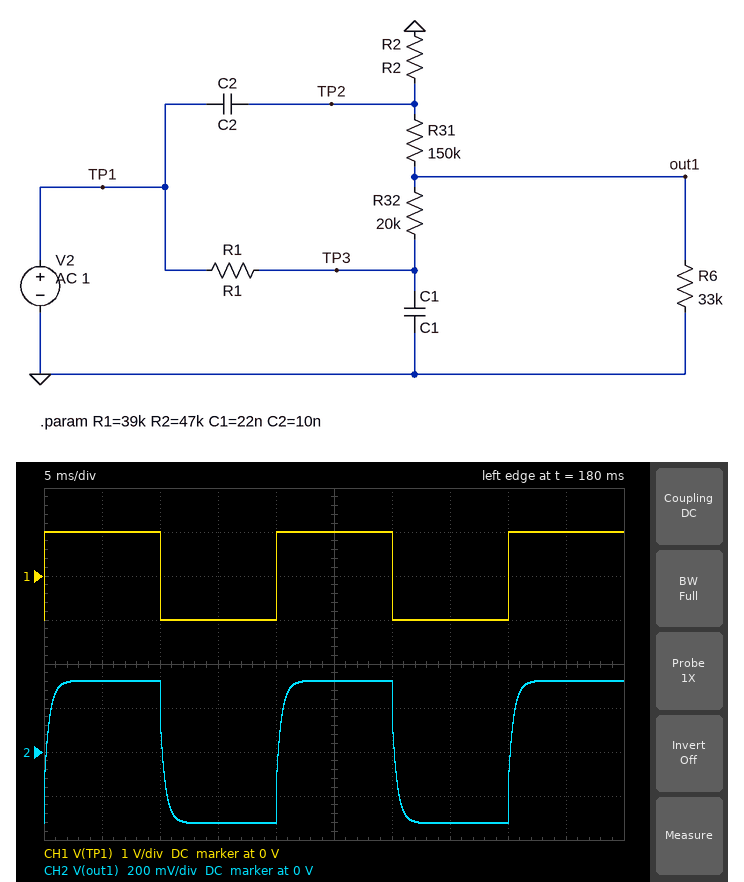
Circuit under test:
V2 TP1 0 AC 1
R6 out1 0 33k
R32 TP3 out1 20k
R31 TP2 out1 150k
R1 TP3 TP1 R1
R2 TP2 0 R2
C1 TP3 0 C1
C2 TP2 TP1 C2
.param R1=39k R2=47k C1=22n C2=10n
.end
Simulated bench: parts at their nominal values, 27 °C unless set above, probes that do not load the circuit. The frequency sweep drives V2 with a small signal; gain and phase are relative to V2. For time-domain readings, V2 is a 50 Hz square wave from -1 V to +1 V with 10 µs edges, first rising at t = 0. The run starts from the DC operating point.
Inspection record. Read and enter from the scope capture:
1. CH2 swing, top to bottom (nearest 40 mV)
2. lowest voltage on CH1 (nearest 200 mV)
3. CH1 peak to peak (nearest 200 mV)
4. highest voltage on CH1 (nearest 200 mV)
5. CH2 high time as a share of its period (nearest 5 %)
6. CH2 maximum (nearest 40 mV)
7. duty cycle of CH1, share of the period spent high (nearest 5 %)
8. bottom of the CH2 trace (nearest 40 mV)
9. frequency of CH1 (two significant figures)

640 mV
-1.0 V
2.0 V
1.0 V
50 %
320 mV
50 %
-320 mV
50 Hz
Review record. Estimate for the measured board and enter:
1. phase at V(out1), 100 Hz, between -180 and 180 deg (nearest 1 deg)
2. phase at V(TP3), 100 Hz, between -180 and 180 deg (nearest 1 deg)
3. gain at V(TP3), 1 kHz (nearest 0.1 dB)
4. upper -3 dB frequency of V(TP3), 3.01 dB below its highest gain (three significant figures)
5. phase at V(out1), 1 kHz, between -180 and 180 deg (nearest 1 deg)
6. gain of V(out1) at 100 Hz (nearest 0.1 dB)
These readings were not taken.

-12 deg
-15 deg
-14.1 dB
375 Hz
-37 deg
-10.1 dB
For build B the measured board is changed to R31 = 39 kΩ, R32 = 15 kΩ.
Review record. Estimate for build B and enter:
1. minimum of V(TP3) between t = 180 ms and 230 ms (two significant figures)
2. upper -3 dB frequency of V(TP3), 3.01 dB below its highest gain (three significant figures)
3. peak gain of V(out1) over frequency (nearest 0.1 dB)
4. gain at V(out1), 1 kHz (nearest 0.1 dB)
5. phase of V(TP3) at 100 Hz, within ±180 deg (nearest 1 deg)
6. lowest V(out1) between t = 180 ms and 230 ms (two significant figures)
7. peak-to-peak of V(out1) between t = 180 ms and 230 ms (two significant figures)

-500 mV
502 Hz
-10.3 dB
-13.5 dB
-11 deg
-310 mV
610 mV
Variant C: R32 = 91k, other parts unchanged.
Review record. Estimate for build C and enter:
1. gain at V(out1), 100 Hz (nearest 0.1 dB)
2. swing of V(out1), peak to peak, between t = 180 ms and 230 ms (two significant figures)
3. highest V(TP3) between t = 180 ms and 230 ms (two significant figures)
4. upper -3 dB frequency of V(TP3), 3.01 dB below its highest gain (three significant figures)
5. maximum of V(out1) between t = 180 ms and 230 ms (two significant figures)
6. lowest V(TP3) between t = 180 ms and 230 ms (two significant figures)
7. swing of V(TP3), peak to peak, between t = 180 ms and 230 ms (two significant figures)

-15.7 dB
360 mV
750 mV
253 Hz
180 mV
-750 mV
1.5 V
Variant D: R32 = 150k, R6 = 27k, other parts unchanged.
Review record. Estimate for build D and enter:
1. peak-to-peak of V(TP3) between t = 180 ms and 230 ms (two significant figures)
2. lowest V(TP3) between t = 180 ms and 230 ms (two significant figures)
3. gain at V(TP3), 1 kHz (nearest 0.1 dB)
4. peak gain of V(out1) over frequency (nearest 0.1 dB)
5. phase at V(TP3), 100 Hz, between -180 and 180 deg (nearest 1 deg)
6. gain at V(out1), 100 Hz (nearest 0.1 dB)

1.6 V
-820 mV
-14.6 dB
-17.6 dB
-23 deg
-19.9 dB
